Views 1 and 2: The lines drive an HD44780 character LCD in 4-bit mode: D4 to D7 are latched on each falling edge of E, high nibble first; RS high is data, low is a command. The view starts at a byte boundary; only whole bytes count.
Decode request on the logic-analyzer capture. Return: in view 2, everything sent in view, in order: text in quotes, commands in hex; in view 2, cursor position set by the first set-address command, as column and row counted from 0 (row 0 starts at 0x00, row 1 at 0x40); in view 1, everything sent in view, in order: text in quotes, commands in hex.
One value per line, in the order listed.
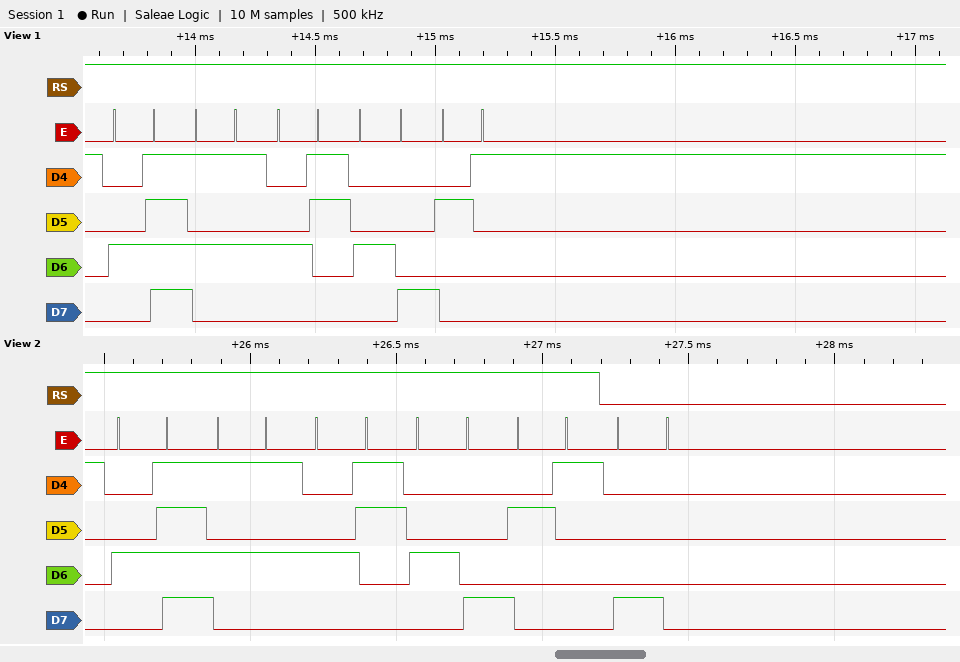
"OUCH!" 0x80
column 0, row 0
"OUCH!"
